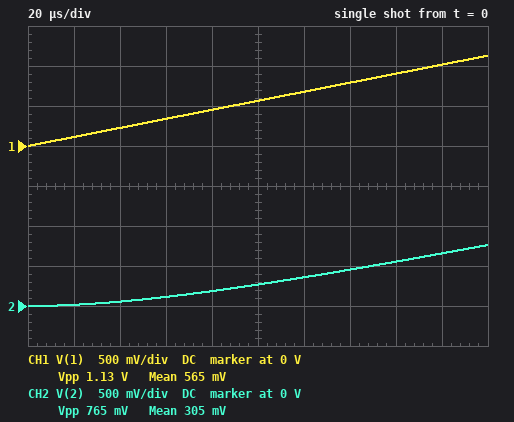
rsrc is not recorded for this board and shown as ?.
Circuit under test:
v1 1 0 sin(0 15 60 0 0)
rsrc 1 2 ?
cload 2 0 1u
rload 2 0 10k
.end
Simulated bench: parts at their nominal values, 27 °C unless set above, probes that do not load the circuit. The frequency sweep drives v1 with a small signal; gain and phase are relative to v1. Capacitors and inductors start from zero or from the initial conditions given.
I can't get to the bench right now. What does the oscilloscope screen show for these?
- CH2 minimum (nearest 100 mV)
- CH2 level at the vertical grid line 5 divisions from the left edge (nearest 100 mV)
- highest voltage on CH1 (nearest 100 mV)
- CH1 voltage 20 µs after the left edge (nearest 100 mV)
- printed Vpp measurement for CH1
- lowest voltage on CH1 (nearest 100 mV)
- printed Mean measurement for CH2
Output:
0 V
300 mV
1.1 V
100 mV
1.13 V
0 V
305 mV
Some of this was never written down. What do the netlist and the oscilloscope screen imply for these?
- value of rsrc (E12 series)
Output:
68 Ω
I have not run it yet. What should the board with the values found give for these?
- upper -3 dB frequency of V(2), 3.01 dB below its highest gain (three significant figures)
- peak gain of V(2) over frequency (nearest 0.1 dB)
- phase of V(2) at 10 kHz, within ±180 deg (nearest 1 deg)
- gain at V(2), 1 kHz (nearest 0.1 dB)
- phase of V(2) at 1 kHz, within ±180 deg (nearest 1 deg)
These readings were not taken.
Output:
2.36 kHz
-0.1 dB
-77 deg
-0.8 dB
-23 deg
